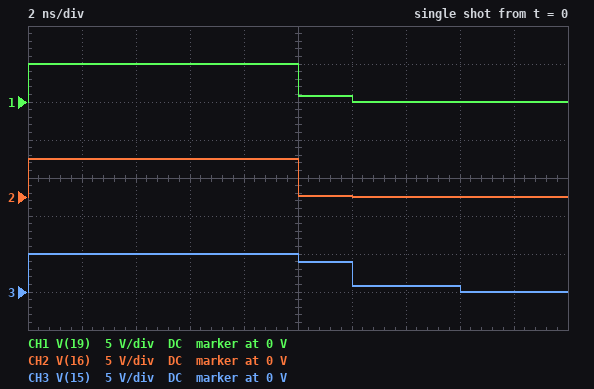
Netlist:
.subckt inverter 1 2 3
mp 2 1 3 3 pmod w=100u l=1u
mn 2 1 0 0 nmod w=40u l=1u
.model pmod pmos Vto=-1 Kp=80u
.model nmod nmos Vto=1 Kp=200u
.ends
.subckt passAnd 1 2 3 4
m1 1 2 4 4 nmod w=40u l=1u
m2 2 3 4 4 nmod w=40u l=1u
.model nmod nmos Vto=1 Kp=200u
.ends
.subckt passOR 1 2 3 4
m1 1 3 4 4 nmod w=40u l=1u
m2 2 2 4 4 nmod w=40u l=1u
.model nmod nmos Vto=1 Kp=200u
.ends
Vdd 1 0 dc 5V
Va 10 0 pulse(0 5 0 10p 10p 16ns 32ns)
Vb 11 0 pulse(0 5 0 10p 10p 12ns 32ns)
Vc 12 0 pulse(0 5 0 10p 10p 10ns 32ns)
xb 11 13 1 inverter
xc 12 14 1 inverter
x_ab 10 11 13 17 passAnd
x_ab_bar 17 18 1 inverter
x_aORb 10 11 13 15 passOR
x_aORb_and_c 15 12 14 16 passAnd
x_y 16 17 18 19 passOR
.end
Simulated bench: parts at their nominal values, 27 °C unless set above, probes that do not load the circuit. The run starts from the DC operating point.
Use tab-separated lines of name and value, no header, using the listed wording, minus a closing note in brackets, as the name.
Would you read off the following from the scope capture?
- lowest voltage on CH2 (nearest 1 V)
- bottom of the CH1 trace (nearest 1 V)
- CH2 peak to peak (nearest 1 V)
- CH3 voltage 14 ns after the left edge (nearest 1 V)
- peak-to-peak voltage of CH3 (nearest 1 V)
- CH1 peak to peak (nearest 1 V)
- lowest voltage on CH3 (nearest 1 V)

lowest voltage on CH2	0 V
bottom of the CH1 trace	0 V
CH2 peak to peak	5 V
CH3 voltage 14 ns after the left edge	1 V
peak-to-peak voltage of CH3	5 V
CH1 peak to peak	5 V
lowest voltage on CH3	0 V
